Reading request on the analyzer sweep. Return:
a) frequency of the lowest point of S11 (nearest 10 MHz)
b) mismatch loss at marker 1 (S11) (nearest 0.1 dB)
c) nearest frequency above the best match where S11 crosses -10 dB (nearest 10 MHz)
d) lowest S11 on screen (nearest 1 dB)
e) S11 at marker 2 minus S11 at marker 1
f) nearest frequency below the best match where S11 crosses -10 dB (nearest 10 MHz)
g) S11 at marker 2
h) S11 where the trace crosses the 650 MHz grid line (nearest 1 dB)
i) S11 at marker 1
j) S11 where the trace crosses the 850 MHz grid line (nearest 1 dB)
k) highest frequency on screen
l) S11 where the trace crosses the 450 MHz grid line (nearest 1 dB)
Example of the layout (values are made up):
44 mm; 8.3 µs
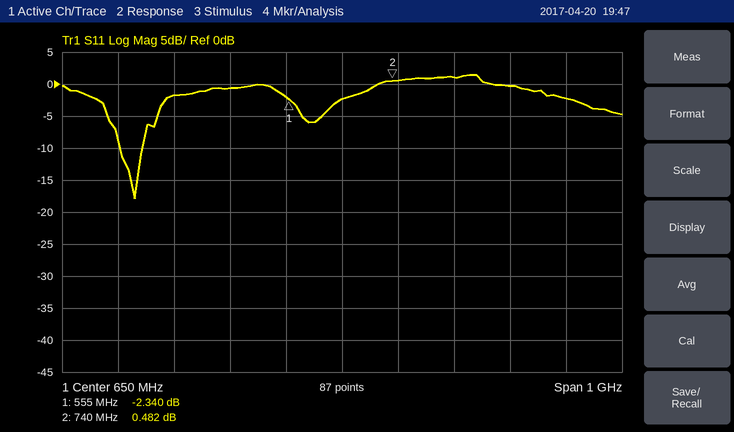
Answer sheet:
280 MHz; 3.8 dB; 290 MHz; -18 dB; 2.822 dB; 250 MHz; 0.482 dB; -2 dB; -2.340 dB; 1 dB; 1.15 GHz; -1 dB
